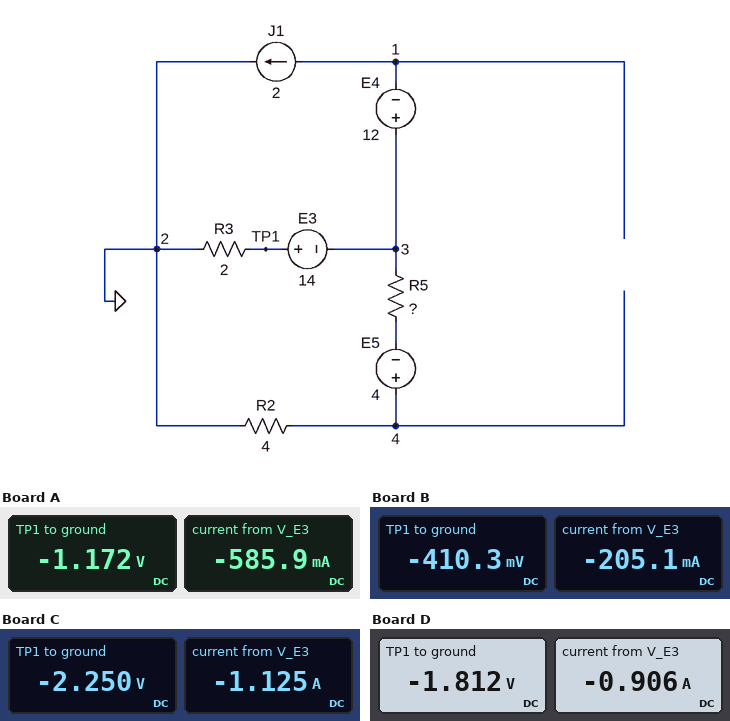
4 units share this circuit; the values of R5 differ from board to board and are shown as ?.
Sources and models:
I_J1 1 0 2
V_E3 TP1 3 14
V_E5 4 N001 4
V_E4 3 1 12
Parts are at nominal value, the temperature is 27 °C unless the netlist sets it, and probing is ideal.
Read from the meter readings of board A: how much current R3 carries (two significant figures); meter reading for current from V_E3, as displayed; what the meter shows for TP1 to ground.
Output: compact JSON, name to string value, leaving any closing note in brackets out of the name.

{"how much current R3 carries": "590 mA", "meter reading for current from V_E3, as displayed": "-585.9 mA", "what the meter shows for TP1 to ground": "-1.172 V"}
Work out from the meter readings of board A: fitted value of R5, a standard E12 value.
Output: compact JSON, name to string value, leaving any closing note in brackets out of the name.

{"fitted value of R5, a standard E12 value": "3.9 Ω"}
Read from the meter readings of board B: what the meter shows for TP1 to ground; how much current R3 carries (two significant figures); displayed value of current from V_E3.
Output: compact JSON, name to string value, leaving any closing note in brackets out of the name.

{"what the meter shows for TP1 to ground": "-410.3 mV", "how much current R3 carries": "210 mA", "displayed value of current from V_E3": "-205.1 mA"}
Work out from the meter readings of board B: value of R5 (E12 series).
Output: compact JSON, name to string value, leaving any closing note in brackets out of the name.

{"value of R5": "1.8 Ω"}
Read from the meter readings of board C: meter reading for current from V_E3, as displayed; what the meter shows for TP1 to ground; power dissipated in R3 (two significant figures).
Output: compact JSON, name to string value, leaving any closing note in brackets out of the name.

{"meter reading for current from V_E3, as displayed": "-1.125 A", "what the meter shows for TP1 to ground": "-2.250 V", "power dissipated in R3": "2.5 W"}
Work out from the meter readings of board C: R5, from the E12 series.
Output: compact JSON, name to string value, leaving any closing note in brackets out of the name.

{"R5, from the E12 series": "10 Ω"}
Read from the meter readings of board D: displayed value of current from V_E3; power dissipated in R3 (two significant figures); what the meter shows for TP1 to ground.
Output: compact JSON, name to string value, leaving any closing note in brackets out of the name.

{"displayed value of current from V_E3": "-0.906 A", "power dissipated in R3": "1.6 W", "what the meter shows for TP1 to ground": "-1.812 V"}
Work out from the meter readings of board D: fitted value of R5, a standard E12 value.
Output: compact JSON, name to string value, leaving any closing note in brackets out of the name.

{"fitted value of R5, a standard E12 value": "6.8 Ω"}
